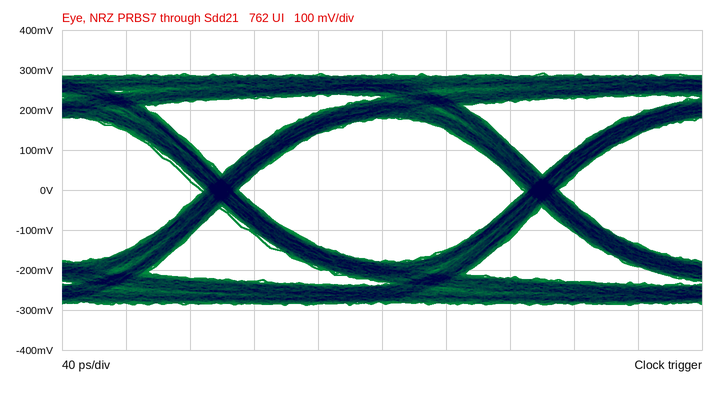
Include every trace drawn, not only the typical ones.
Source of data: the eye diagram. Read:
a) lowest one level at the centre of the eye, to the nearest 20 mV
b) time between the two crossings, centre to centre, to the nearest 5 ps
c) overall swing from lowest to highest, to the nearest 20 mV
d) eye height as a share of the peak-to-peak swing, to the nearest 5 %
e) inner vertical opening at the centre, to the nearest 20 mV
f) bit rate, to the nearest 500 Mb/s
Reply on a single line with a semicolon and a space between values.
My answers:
180 mV; 200 ps; 580 mV; 60 %; 360 mV; 5.0 Gb/s
